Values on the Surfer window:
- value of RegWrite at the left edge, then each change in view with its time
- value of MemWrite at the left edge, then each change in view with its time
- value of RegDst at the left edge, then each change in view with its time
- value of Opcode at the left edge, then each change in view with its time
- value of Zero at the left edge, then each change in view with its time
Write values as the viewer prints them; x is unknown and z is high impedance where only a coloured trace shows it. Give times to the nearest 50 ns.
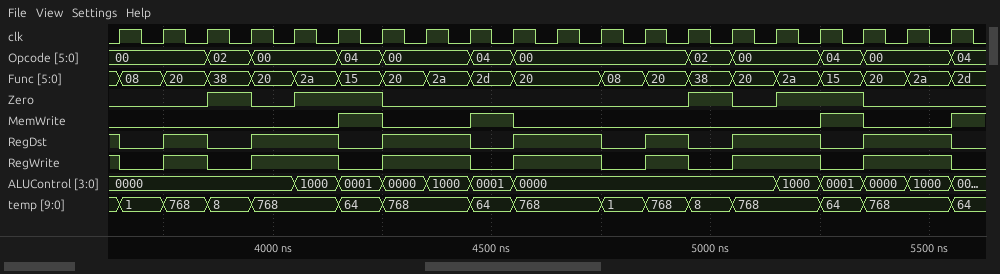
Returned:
1, 0 at 3650 ns, 1 at 3750 ns, 0 at 3850 ns, 1 at 3950 ns, 0 at 4150 ns, 1 at 4250 ns, 0 at 4450 ns, 1 at 4550 ns, 0 at 4750 ns, 1 at 4850 ns, 0 at 4950 ns, 1 at 5050 ns, 0 at 5250 ns, 1 at 5350 ns, 0 at 5550 ns
0, 1 at 4150 ns, 0 at 4250 ns, 1 at 4450 ns, 0 at 4550 ns, 1 at 5250 ns, 0 at 5350 ns, 1 at 5550 ns
1, 0 at 3650 ns, 1 at 3750 ns, 0 at 3850 ns, 1 at 3950 ns, 0 at 4150 ns, 1 at 4250 ns, 0 at 4450 ns, 1 at 4550 ns, 0 at 4750 ns, 1 at 4850 ns, 0 at 4950 ns, 1 at 5050 ns, 0 at 5250 ns, 1 at 5350 ns, 0 at 5550 ns
00, 02 at 3850 ns, 00 at 3950 ns, 04 at 4150 ns, 00 at 4250 ns, 04 at 4450 ns, 00 at 4550 ns, 02 at 4950 ns, 00 at 5050 ns, 04 at 5250 ns, 00 at 5350 ns, 04 at 5550 ns
0, 1 at 3850 ns, 0 at 3950 ns, 1 at 4050 ns, 0 at 4250 ns, 1 at 4950 ns, 0 at 5050 ns, 1 at 5150 ns, 0 at 5350 ns
